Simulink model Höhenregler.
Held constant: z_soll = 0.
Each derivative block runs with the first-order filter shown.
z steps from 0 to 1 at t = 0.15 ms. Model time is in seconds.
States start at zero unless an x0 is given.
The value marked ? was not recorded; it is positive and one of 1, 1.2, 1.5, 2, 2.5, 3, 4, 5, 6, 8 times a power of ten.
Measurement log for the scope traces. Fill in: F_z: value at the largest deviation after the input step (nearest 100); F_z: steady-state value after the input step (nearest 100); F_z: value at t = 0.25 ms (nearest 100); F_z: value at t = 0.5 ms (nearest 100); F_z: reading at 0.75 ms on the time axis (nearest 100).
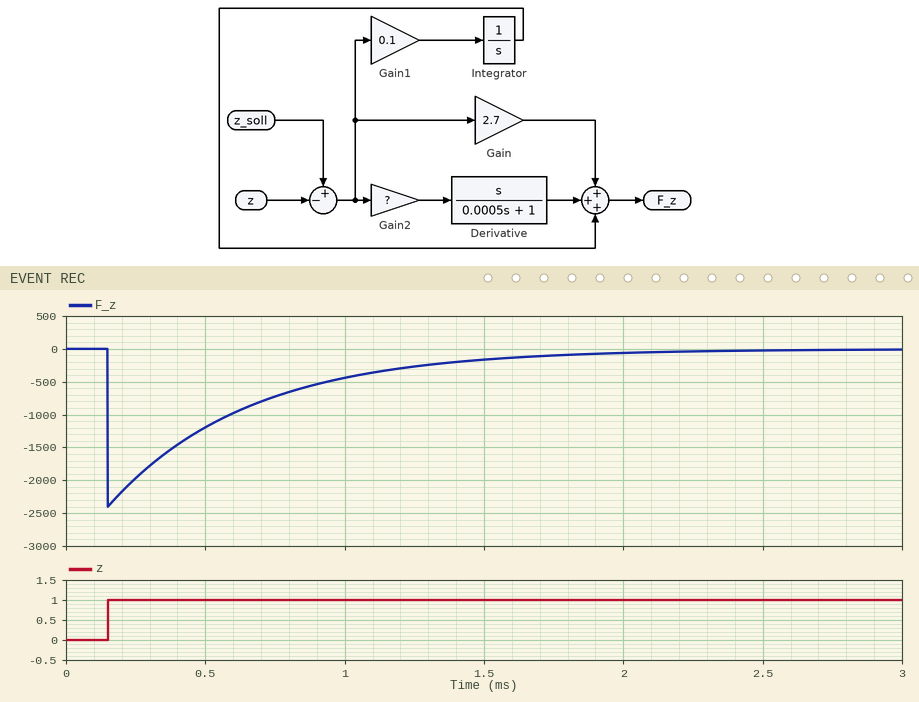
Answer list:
-2400
0
-2000
-1200
-700
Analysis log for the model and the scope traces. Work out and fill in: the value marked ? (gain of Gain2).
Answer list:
1.2
